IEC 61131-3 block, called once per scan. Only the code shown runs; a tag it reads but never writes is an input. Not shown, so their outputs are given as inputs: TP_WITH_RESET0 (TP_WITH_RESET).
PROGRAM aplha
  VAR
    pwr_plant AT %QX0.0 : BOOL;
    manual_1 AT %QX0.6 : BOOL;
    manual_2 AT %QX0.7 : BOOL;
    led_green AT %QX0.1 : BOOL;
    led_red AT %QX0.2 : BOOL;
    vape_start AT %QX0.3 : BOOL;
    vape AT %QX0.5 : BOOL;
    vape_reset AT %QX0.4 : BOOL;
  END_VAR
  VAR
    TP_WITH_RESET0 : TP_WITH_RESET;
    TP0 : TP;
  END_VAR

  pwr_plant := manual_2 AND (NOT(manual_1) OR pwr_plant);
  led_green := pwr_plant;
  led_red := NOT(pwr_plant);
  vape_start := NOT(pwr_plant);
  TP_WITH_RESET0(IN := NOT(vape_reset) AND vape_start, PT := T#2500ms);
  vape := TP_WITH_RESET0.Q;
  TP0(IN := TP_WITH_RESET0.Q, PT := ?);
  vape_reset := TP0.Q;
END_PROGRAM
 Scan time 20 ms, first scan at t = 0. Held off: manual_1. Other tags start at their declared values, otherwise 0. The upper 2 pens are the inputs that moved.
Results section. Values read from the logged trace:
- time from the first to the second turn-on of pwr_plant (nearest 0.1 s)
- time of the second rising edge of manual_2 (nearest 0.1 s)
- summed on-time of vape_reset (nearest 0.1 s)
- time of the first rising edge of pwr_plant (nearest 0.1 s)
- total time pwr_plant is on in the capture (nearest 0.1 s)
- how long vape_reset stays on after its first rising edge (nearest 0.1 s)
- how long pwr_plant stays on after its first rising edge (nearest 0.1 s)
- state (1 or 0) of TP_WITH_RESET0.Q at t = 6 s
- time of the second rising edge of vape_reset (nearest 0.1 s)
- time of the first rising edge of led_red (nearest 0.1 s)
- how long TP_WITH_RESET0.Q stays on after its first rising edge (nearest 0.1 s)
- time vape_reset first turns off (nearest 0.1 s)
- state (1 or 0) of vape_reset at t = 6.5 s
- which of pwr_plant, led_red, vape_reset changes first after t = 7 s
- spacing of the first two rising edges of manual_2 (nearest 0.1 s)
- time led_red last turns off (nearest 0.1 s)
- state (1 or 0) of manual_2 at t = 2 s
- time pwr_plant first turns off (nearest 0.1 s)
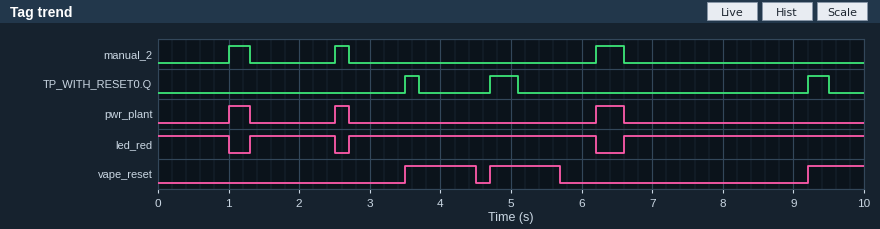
1.5 s
2.5 s
2.8 s
1.0 s
0.9 s
1.0 s
0.3 s
0
4.7 s
1.3 s
0.2 s
4.5 s
0
vape_reset
1.5 s
6.2 s
0
1.3 s
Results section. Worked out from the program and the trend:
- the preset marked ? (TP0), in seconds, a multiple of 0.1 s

1.0 s
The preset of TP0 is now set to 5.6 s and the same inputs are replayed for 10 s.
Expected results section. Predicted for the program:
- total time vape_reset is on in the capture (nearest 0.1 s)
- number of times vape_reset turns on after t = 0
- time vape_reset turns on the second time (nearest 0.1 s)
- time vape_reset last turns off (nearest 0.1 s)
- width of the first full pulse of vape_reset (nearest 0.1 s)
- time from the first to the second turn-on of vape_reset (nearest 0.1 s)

6.4 s
2
9.2 s
9.1 s
5.6 s
5.7 s
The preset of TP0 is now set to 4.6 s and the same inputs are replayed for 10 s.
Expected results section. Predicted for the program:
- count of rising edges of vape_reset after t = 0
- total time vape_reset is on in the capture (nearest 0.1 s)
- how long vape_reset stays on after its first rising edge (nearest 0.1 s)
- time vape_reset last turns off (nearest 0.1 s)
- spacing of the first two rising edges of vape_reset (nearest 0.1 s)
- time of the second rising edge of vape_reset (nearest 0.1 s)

2
5.4 s
4.6 s
8.1 s
5.7 s
9.2 s
